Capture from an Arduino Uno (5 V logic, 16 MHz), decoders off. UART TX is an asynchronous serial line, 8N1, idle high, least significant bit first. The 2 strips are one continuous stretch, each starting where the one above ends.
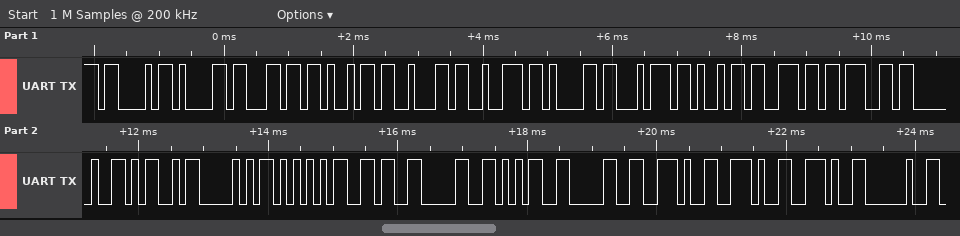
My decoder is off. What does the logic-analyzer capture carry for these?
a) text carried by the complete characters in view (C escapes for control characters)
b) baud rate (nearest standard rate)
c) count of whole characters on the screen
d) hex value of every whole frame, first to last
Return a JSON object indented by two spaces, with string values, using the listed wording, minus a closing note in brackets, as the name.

{
  "text carried by the complete characters in view": "\"Calibrating MPU6050... \"",
  "baud rate": "9600 baud",
  "count of whole characters on the screen": "23",
  "hex value of every whole frame, first to last": "43 61 6C 69 62 72 61 74 69 6E 67 20 4D 50 55 36 30 35 30 2E 2E 2E 20"
}
